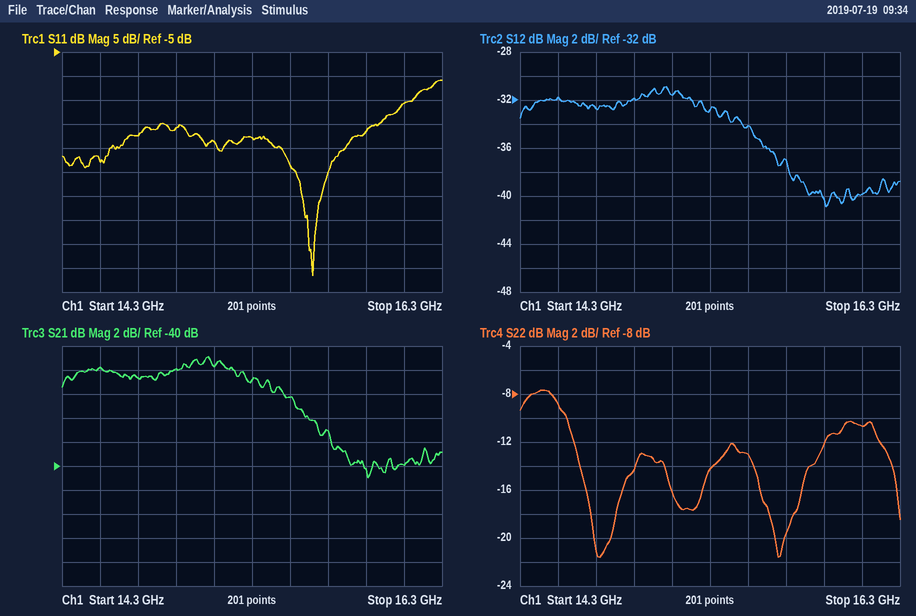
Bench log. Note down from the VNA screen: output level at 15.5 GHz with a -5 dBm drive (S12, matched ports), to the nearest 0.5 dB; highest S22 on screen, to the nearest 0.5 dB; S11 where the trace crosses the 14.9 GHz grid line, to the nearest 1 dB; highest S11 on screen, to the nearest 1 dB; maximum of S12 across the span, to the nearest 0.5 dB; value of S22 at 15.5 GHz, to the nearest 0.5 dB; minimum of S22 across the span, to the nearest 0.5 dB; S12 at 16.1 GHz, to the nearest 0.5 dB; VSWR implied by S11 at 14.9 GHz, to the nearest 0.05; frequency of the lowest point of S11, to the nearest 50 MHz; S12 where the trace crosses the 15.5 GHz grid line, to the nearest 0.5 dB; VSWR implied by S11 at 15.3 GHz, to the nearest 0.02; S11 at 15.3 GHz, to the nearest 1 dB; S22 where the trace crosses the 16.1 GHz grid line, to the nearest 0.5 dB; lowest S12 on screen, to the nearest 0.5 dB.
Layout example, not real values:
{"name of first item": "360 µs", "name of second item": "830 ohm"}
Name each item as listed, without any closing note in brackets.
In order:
{"output level at 15.5 GHz with a -5 dBm drive (S12, matched ports), to the nearest 0.5 dB": "-39.0 dBm", "highest S22 on screen, to the nearest 0.5 dB": "-7.5 dB", "S11 where the trace crosses the 14.9 GHz grid line, to the nearest 1 dB": "-21 dB", "highest S11 on screen, to the nearest 1 dB": "-11 dB", "maximum of S12 across the span, to the nearest 0.5 dB": "-31.0 dB", "value of S22 at 15.5 GHz, to the nearest 0.5 dB": "-13.0 dB", "minimum of S22 across the span, to the nearest 0.5 dB": "-21.5 dB", "S12 at 16.1 GHz, to the nearest 0.5 dB": "-40.0 dB", "VSWR implied by S11 at 14.9 GHz, to the nearest 0.05": "1.20", "frequency of the lowest point of S11, to the nearest 50 MHz": "15.60 GHz", "S12 where the trace crosses the 15.5 GHz grid line, to the nearest 0.5 dB": "-34.0 dB", "VSWR implied by S11 at 15.3 GHz, to the nearest 0.02": "1.16", "S11 at 15.3 GHz, to the nearest 1 dB": "-23 dB", "S22 where the trace crosses the 16.1 GHz grid line, to the nearest 0.5 dB": "-10.5 dB", "lowest S12 on screen, to the nearest 0.5 dB": "-41.0 dB"}
